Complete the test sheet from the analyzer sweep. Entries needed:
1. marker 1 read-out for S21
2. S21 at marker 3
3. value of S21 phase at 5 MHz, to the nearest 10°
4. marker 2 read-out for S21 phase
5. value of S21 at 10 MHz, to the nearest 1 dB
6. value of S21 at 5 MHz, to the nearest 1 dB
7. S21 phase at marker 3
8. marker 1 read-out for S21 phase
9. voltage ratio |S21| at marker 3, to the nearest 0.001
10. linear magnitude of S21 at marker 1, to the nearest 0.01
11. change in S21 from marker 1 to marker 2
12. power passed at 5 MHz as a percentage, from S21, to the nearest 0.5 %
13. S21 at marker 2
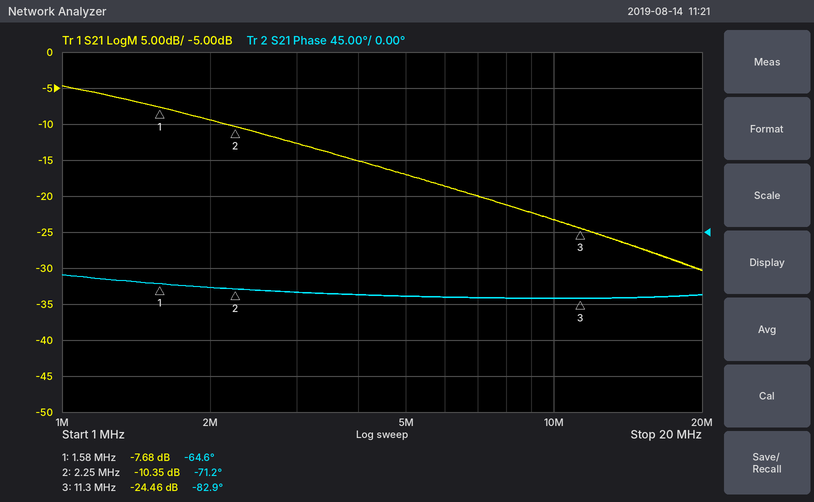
-7.68 dB
-24.46 dB
-80°
-71.2°
-23 dB
-17 dB
-82.9°
-64.6°
0.060
0.41
-2.67 dB
2.0 %
-10.35 dB
